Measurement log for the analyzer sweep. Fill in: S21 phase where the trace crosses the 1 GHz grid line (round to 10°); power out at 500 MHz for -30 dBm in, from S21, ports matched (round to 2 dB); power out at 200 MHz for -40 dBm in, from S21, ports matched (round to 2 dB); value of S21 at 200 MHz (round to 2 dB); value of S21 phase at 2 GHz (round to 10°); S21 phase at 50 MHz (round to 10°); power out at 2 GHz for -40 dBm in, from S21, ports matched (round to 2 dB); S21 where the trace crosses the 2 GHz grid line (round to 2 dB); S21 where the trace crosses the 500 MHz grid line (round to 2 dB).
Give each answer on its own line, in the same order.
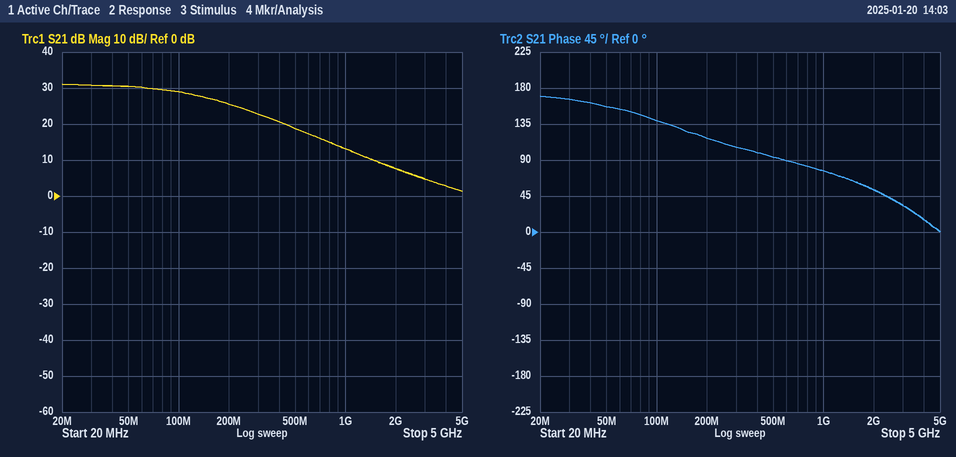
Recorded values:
80°
-12 dBm
-14 dBm
26 dB
50°
160°
-32 dBm
8 dB
18 dB
